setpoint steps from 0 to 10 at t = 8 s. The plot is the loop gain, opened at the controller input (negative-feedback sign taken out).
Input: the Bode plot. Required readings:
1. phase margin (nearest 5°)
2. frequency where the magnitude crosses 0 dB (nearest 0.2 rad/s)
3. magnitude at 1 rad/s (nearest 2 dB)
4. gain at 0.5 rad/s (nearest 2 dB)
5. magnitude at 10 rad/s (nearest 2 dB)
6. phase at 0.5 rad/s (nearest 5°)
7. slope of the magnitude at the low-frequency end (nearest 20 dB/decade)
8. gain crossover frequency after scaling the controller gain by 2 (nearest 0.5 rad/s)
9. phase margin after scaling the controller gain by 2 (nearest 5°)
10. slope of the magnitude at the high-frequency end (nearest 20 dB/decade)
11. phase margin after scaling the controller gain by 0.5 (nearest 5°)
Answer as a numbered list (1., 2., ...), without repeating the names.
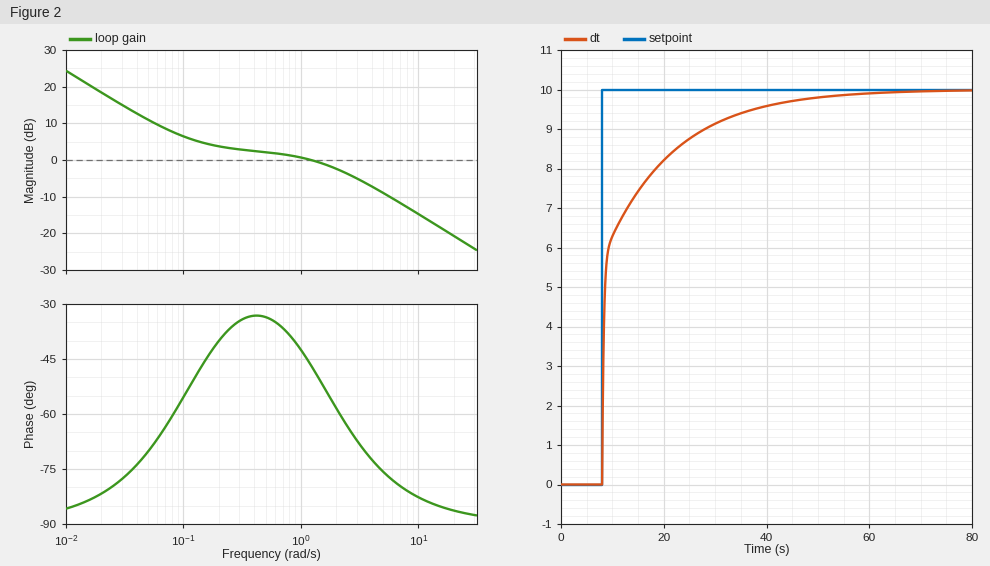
1. 135°
2. 1.2 rad/s
3. 0 dB
4. 2 dB
5. -14 dB
6. -35°
7. -20 dB/decade
8. 3.5 rad/s
9. 110°
10. -20 dB/decade
11. 125°
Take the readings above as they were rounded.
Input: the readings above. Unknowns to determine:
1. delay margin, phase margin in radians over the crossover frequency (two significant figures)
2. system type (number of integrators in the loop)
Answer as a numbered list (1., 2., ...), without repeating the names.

1. 2.0 s
2. 1
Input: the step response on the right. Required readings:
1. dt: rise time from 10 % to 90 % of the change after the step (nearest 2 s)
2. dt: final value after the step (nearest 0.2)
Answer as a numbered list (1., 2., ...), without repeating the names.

1. 20 s
2. 10.0
